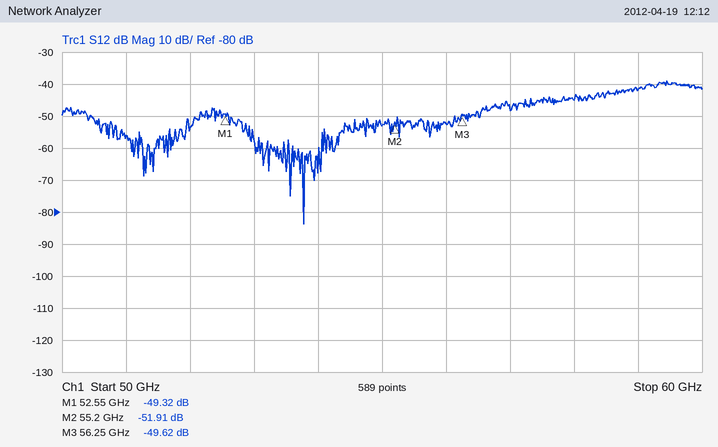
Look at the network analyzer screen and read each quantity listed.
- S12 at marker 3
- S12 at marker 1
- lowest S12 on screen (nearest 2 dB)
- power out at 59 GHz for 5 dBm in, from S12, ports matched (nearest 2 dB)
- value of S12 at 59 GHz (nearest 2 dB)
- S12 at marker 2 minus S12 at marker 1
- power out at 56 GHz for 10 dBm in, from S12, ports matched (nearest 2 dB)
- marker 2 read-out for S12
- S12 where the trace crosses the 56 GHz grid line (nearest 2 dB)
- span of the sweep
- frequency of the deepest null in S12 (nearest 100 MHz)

-49.62 dB
-49.32 dB
-84 dB
-36 dBm
-42 dB
-2.59 dB
-42 dBm
-51.91 dB
-52 dB
10 GHz
53.8 GHz
